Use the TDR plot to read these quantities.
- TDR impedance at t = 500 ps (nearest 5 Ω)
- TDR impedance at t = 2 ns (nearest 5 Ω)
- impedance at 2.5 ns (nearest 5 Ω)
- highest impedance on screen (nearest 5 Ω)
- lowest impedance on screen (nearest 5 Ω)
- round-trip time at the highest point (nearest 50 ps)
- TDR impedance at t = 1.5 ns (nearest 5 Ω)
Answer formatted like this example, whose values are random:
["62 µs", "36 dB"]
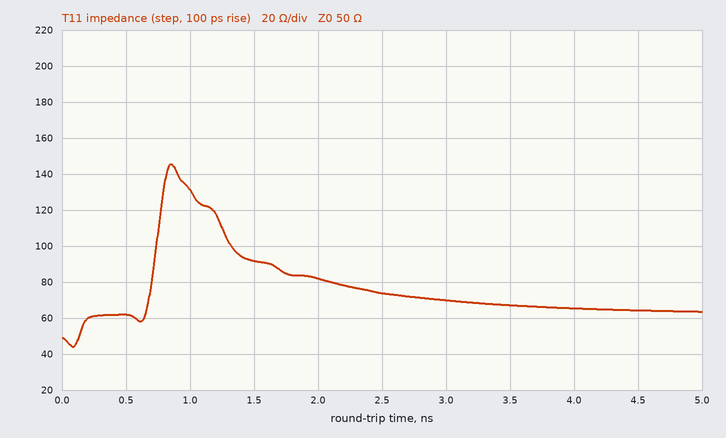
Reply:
["60 Ω", "80 Ω", "75 Ω", "145 Ω", "45 Ω", "850 ps", "90 Ω"]
